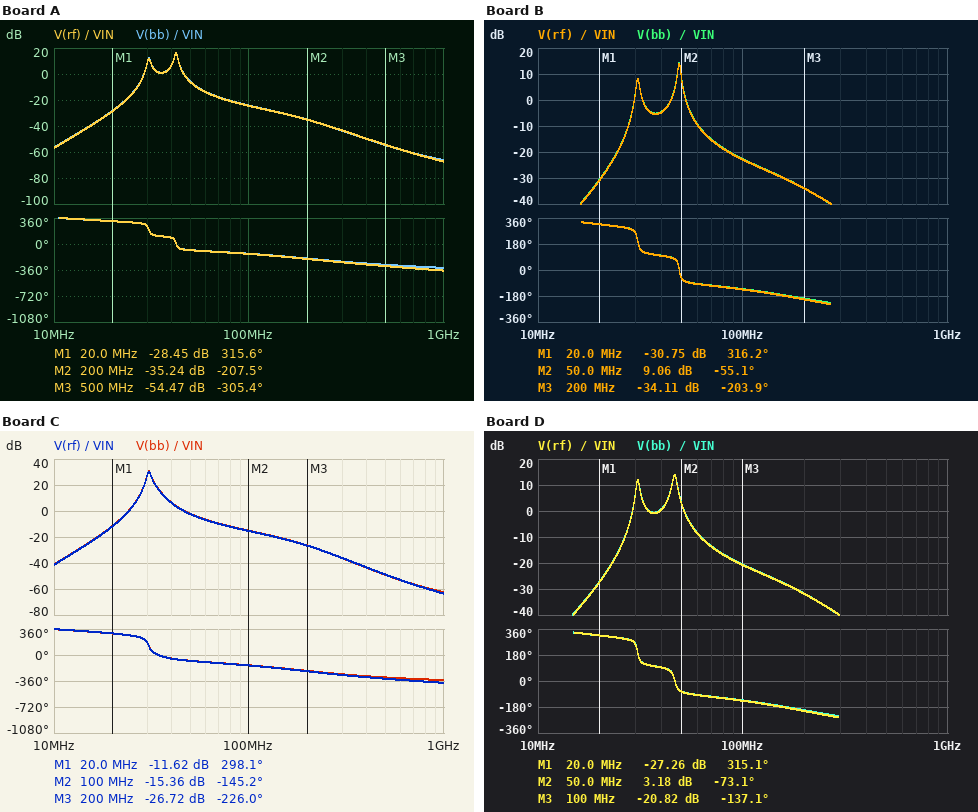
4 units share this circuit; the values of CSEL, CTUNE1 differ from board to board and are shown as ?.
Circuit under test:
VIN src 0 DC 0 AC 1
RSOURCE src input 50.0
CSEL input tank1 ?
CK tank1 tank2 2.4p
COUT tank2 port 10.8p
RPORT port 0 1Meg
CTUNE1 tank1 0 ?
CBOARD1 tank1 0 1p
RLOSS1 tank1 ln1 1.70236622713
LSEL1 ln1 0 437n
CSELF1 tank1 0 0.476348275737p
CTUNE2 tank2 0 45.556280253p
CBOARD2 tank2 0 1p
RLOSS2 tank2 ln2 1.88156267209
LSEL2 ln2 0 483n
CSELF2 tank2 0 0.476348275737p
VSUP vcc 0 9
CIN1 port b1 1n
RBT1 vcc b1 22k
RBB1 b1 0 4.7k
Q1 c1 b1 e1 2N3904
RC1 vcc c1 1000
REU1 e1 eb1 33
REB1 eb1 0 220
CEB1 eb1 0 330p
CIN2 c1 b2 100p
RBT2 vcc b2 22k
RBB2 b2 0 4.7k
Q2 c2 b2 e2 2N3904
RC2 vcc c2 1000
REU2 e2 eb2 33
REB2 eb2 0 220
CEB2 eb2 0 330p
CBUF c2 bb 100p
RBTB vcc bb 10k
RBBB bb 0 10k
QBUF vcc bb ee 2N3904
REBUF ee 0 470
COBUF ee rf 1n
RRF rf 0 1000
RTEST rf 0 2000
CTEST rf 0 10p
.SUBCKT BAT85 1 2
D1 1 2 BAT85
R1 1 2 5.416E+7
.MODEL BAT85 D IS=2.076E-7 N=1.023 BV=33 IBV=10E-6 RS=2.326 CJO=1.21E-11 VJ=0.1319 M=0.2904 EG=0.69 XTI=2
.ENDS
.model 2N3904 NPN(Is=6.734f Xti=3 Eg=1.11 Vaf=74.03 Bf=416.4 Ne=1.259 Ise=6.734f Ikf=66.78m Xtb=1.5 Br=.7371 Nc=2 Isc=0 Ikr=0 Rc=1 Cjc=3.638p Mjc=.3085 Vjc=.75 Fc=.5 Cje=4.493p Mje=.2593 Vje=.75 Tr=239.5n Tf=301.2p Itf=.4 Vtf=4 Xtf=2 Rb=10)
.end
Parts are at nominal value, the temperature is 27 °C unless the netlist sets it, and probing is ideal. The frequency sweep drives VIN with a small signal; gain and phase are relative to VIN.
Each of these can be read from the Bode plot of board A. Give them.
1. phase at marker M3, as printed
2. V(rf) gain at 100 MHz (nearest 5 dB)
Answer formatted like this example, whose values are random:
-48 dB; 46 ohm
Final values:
-305.4 deg; -25 dB
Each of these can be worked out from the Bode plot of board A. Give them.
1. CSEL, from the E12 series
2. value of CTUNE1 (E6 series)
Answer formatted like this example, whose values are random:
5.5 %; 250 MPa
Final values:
6.8 pF; 22 pF
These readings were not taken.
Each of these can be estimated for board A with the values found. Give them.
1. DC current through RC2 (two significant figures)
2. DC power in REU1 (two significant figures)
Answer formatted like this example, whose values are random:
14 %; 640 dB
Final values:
3.2 mA; 340 µW
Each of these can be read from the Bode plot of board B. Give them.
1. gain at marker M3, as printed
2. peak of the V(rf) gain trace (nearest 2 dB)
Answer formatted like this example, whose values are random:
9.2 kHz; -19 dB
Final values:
-34.11 dB; 14 dB
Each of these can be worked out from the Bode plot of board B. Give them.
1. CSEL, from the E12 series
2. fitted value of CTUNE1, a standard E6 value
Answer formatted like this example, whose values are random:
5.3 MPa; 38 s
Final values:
5.6 pF; 15 pF
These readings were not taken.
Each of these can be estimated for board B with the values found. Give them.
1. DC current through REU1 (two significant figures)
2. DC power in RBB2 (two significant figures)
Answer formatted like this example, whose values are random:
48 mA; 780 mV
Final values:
3.2 mA; 480 µW
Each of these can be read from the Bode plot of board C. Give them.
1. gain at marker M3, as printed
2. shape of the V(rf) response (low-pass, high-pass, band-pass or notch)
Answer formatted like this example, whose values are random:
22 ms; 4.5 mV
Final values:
-26.72 dB; band-pass
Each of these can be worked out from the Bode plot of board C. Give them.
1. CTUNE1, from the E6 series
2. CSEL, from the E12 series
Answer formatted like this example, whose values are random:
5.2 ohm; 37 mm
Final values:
15 pF; 39 pF
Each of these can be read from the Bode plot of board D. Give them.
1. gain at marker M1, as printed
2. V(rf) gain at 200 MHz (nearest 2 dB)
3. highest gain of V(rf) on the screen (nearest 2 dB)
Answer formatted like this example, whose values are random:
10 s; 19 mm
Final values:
-27.26 dB; -32 dB; 14 dB
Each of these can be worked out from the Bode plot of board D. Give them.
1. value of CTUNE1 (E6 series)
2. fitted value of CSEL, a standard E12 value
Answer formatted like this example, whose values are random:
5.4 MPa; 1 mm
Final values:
15 pF; 8.2 pF
